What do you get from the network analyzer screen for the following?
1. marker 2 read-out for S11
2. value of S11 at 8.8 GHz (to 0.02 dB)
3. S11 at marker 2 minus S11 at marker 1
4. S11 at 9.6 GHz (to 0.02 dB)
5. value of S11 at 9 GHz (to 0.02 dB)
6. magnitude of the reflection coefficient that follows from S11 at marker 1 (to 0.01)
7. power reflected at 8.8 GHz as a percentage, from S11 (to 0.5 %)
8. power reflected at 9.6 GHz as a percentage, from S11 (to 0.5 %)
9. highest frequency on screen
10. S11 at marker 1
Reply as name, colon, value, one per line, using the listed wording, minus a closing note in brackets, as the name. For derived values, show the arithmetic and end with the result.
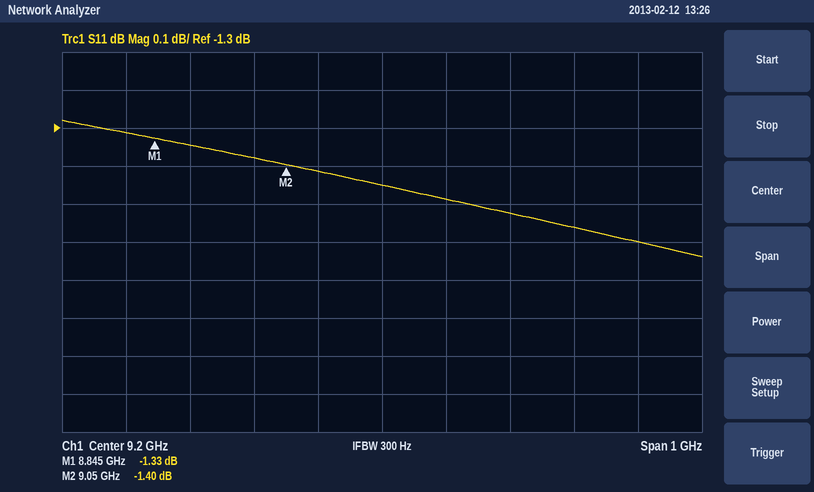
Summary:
marker 2 read-out for S11: -1.40 dB
value of S11 at 8.8 GHz: -1.32 dB
S11 at marker 2 minus S11 at marker 1: -1.4 − (-1.33) = -0.07 dB
S11 at 9.6 GHz: -1.60 dB
value of S11 at 9 GHz: -1.38 dB
magnitude of the reflection coefficient that follows from S11 at marker 1: 10^(-1.33/20) ≈ 0.86
power reflected at 8.8 GHz as a percentage, from S11: 10^(-1.32/10) ≈ 73.8 %, so 74.0 % to the nearest 0.5 %
power reflected at 9.6 GHz as a percentage, from S11: 10^(-1.6/10) ≈ 69.2 %, so 69.0 % to the nearest 0.5 %
highest frequency on screen: 9.7 GHz
S11 at marker 1: -1.33 dB
